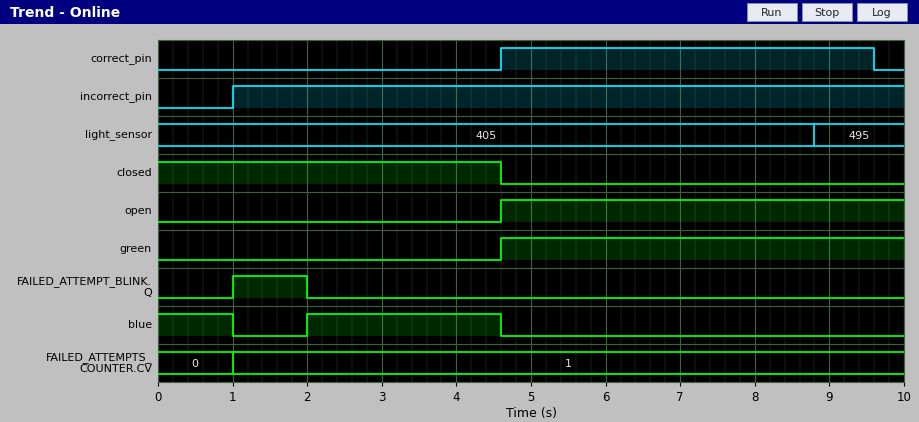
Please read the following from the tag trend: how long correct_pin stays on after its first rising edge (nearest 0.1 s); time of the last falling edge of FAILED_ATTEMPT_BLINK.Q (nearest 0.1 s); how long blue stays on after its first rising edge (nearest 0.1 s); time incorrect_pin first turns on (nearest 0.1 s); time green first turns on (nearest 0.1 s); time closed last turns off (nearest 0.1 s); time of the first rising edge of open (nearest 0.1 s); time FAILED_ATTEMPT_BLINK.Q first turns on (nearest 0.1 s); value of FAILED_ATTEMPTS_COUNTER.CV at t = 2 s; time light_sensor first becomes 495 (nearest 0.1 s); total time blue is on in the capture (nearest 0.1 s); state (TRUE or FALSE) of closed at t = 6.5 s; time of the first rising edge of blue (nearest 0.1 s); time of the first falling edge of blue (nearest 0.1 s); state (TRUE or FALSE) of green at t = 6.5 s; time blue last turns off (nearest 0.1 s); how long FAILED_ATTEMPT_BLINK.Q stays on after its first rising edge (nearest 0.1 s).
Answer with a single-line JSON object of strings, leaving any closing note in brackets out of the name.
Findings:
{"how long correct_pin stays on after its first rising edge": "5.0 s", "time of the last falling edge of FAILED_ATTEMPT_BLINK.Q": "2.0 s", "how long blue stays on after its first rising edge": "2.6 s", "time incorrect_pin first turns on": "1.0 s", "time green first turns on": "4.6 s", "time closed last turns off": "4.6 s", "time of the first rising edge of open": "4.6 s", "time FAILED_ATTEMPT_BLINK.Q first turns on": "1.0 s", "value of FAILED_ATTEMPTS_COUNTER.CV at t = 2 s": "1", "time light_sensor first becomes 495": "8.8 s", "total time blue is on in the capture": "3.6 s", "state (TRUE or FALSE) of closed at t = 6.5 s": "FALSE", "time of the first rising edge of blue": "2.0 s", "time of the first falling edge of blue": "1.0 s", "state (TRUE or FALSE) of green at t = 6.5 s": "TRUE", "time blue last turns off": "4.6 s", "how long FAILED_ATTEMPT_BLINK.Q stays on after its first rising edge": "1.0 s"}
